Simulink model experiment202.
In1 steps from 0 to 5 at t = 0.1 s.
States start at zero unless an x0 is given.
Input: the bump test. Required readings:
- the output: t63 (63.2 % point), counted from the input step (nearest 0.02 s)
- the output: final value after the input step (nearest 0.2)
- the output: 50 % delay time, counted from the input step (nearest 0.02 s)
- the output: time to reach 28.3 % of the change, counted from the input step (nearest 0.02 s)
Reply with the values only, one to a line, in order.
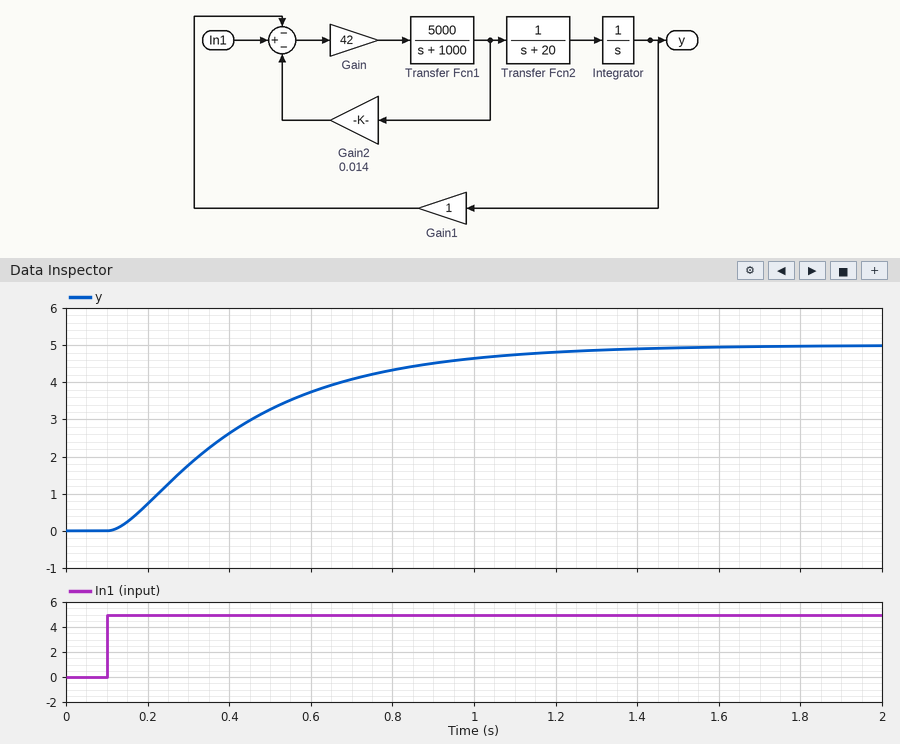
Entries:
0.38 s
5.0
0.28 s
0.16 s
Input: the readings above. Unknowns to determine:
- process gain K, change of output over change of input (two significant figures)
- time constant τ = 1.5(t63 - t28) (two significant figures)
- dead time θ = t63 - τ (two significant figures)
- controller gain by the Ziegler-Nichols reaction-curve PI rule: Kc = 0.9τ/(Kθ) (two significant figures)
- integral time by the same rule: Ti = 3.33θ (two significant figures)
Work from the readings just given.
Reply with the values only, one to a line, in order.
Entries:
1.0
0.33 s
0.050 s
5.9
0.17 s
